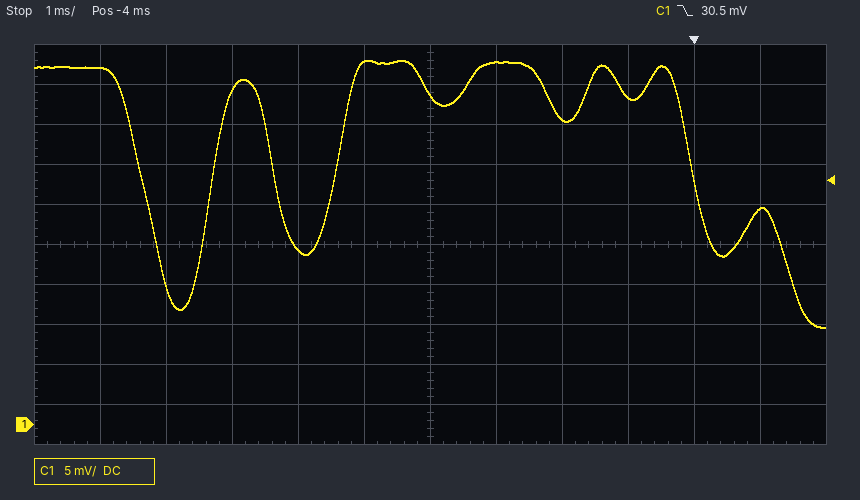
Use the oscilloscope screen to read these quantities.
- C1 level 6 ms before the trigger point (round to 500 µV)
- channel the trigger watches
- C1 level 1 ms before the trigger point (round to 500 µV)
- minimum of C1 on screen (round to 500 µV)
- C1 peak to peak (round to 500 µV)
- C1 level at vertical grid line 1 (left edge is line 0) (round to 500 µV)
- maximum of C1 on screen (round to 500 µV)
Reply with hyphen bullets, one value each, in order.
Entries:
- 22.0 mV
- C1
- 41.0 mV
- 12.0 mV
- 33.5 mV
- 44.5 mV
- 45.5 mV
